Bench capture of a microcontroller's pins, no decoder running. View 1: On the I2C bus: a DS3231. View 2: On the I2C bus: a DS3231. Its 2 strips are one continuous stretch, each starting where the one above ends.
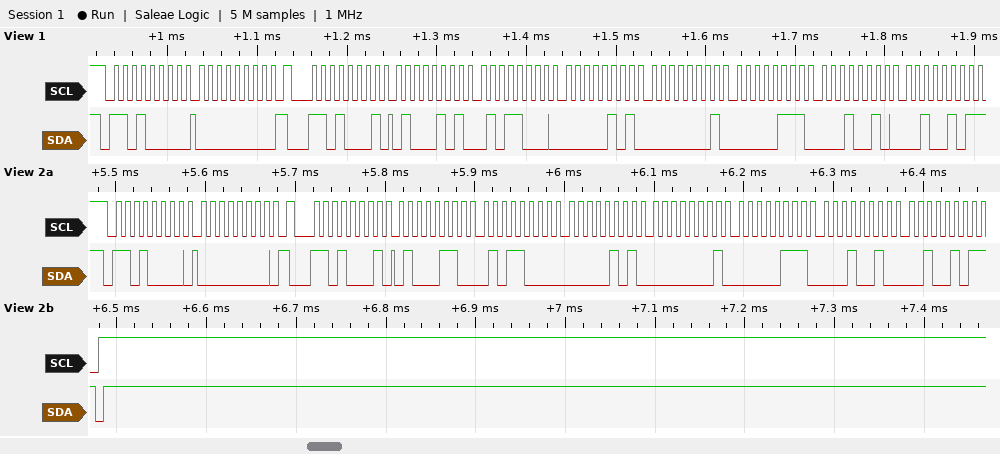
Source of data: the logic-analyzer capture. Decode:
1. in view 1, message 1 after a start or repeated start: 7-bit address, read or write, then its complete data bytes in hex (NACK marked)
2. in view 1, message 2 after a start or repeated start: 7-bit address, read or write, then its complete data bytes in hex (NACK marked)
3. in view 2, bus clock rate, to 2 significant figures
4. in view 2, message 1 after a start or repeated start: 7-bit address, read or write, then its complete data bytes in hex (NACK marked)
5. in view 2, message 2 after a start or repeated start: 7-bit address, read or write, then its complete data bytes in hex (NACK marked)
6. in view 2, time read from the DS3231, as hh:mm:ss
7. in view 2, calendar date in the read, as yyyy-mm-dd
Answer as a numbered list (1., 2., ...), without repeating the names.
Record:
1. 0x68 write: 00
2. 0x68 read: 45 58 05 01 07 12 25 NACK
3. 100 kHz
4. 0x68 write: 00
5. 0x68 read: 46 58 05 01 07 12 25 NACK
6. 05:58:46
7. 2025-12-07
